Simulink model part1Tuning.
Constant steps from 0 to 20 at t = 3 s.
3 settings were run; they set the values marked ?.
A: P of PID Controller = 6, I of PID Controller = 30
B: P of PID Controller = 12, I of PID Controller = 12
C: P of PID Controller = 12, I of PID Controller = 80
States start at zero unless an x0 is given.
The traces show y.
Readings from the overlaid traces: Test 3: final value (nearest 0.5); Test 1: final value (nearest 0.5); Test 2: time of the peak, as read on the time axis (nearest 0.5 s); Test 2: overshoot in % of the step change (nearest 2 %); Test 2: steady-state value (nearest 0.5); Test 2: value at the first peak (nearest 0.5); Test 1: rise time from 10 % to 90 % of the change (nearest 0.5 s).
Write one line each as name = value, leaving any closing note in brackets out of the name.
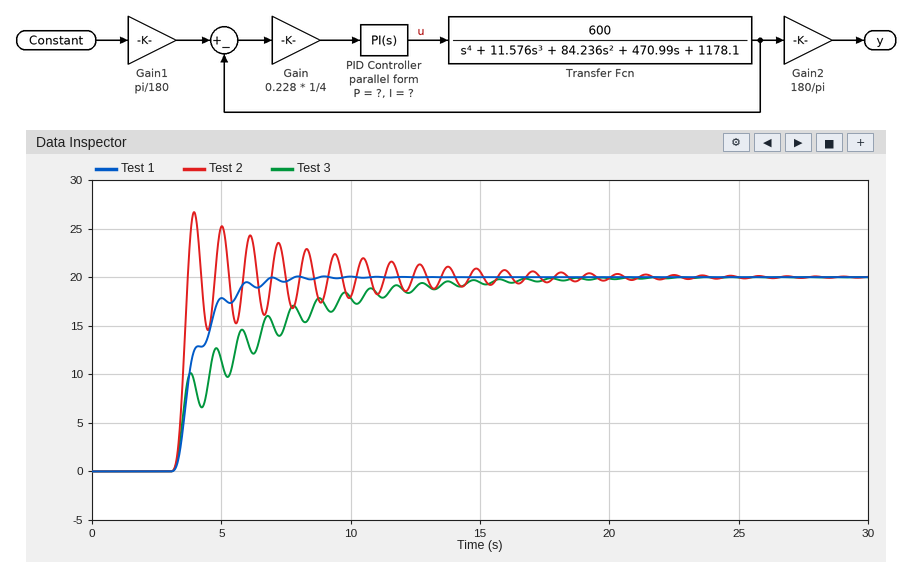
Test 3: final value = 20.0
Test 1: final value = 20.0
Test 2: time of the peak, as read on the time axis = 4.0 s
Test 2: overshoot in % of the step change = 34 %
Test 2: steady-state value = 20.0
Test 2: value at the first peak = 26.5
Test 1: rise time from 10 % to 90 % of the change = 2.0 s
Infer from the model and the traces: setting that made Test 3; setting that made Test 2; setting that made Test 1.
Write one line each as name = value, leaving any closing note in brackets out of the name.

setting that made Test 3 = B
setting that made Test 2 = C
setting that made Test 1 = A
